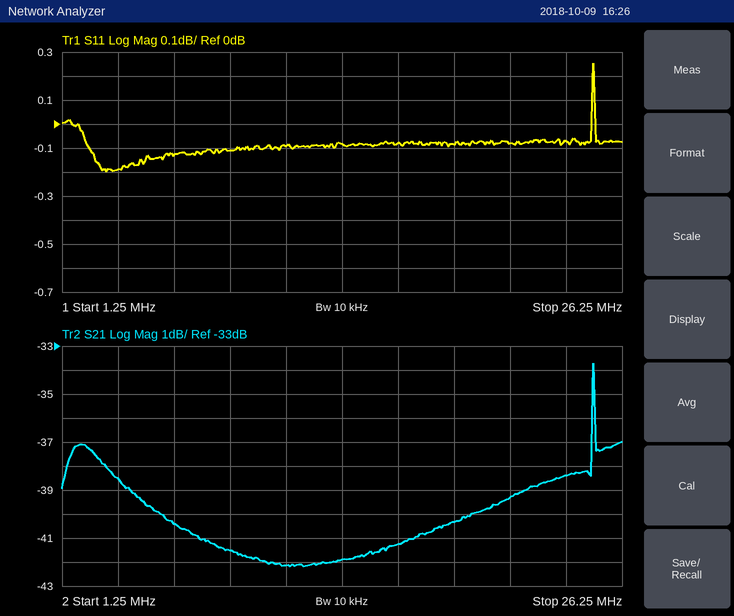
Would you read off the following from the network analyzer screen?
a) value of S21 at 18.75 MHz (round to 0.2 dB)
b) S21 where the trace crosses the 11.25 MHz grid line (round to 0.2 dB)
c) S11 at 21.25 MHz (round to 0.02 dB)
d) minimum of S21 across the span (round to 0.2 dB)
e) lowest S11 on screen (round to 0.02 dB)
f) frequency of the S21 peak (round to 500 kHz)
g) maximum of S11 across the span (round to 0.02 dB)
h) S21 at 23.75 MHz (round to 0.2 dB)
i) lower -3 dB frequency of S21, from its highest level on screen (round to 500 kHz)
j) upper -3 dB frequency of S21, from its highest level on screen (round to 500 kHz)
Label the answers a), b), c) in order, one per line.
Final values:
a) -40.4 dB
b) -42.2 dB
c) -0.08 dB
d) -42.2 dB
e) -0.20 dB
f) 25.0 MHz
g) 0.26 dB
h) -38.4 dB
i) 25.0 MHz
j) 25.0 MHz
